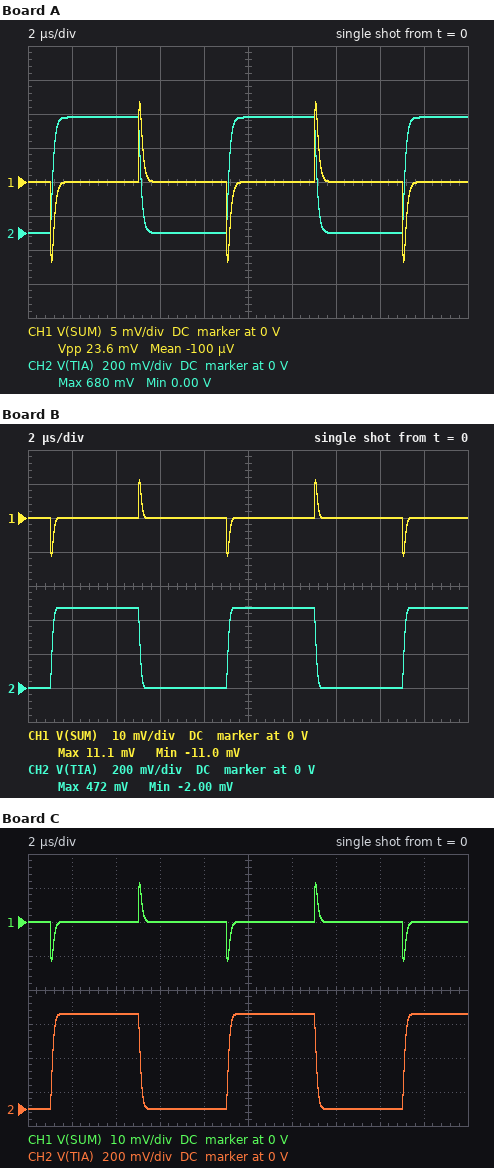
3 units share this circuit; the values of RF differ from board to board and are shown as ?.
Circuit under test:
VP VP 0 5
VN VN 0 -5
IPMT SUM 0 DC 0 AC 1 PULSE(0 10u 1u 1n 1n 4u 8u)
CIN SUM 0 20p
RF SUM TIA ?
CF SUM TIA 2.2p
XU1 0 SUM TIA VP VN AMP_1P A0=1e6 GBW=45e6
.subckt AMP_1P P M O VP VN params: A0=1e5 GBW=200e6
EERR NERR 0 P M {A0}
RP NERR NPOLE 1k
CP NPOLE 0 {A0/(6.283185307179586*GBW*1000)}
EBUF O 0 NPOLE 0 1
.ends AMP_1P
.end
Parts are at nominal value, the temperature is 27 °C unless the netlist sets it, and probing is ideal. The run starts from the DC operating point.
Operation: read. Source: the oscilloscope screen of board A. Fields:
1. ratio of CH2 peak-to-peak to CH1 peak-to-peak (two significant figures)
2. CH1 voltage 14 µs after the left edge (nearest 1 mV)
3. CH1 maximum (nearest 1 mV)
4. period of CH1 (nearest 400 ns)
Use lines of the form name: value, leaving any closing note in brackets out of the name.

ratio of CH2 peak-to-peak to CH1 peak-to-peak: 29
CH1 voltage 14 µs after the left edge: 0 V
CH1 maximum: 12 mV
period of CH1: 8.0 µs
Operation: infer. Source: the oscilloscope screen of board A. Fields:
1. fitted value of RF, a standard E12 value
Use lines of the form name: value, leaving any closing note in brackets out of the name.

fitted value of RF, a standard E12 value: 68 kΩ
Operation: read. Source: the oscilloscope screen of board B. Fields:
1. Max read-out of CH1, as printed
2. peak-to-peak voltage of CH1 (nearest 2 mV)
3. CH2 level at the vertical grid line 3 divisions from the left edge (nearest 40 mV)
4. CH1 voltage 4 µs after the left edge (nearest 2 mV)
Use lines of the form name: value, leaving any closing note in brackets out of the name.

Max read-out of CH1, as printed: 11.1 mV
peak-to-peak voltage of CH1: 22 mV
CH2 level at the vertical grid line 3 divisions from the left edge: 0 V
CH1 voltage 4 µs after the left edge: 0 V
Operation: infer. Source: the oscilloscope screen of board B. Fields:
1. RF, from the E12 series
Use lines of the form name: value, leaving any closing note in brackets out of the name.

RF, from the E12 series: 47 kΩ
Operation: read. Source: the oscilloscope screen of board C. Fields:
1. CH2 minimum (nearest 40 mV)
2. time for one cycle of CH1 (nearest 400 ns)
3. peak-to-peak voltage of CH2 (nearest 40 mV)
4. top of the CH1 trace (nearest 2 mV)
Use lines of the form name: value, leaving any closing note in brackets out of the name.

CH2 minimum: 0 V
time for one cycle of CH1: 8.0 µs
peak-to-peak voltage of CH2: 560 mV
top of the CH1 trace: 12 mV
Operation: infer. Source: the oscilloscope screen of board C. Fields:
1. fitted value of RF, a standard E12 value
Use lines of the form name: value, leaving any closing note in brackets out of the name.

fitted value of RF, a standard E12 value: 56 kΩ
